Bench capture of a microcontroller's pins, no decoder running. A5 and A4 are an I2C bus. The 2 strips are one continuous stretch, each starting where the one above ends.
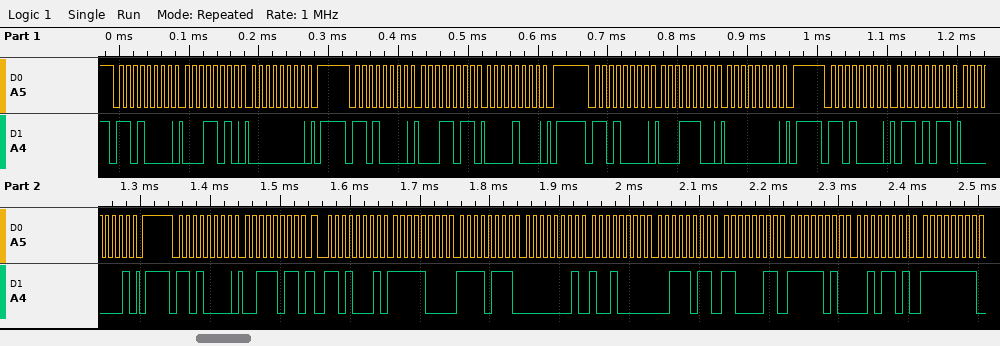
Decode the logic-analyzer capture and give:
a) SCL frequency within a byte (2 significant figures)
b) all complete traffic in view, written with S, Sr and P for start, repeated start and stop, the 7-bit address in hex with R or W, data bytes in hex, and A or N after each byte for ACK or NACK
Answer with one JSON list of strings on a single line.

["100 kHz", "S 68W A 1A A 00 A P S 68W A 1B A 08 A P S 68W A 1C A 00 A P S 68W A 6B A 01 A P S 68W A 3B A Sr 68R A F8 A F7 A 01 A 90 A 3B A C3 A FA A 2D A FF A"]
